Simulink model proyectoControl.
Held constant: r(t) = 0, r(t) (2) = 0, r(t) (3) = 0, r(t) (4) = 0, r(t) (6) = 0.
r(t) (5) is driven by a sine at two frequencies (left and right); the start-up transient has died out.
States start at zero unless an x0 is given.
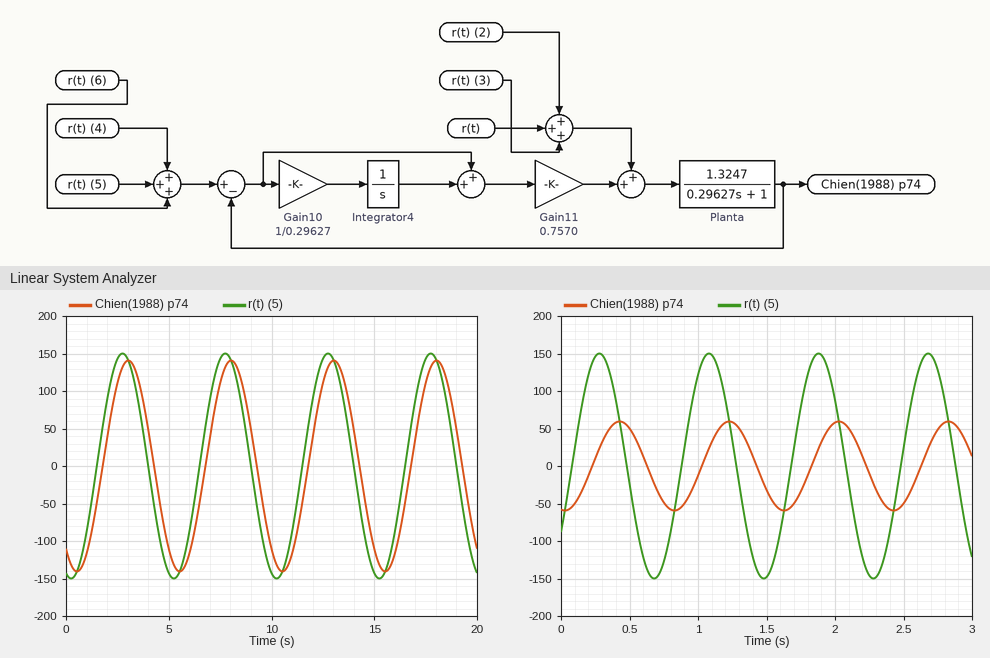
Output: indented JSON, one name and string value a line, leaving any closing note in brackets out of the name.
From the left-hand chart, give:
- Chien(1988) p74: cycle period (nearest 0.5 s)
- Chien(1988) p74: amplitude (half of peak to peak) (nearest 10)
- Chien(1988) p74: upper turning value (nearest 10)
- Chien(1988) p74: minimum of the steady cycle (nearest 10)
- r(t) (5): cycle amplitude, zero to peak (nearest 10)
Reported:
{
  "Chien(1988) p74: cycle period": "5.0 s",
  "Chien(1988) p74: amplitude (half of peak to peak)": "140",
  "Chien(1988) p74: upper turning value": "140",
  "Chien(1988) p74: minimum of the steady cycle": "-140",
  "r(t) (5): cycle amplitude, zero to peak": "150"
}
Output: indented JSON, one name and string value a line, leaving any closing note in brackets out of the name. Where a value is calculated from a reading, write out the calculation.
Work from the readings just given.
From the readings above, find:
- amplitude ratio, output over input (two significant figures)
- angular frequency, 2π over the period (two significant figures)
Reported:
{
  "amplitude ratio, output over input": "140 / 150 = 0.93",
  "angular frequency, 2π over the period": "2π / 5 = 1.3 rad/s"
}
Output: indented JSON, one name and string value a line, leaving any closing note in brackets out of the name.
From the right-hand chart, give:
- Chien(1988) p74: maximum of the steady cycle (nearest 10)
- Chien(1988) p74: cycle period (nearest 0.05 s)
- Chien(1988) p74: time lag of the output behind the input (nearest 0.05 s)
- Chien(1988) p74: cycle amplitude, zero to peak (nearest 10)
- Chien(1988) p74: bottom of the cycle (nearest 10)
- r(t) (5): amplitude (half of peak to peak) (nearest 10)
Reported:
{
  "Chien(1988) p74: maximum of the steady cycle": "60",
  "Chien(1988) p74: cycle period": "0.80 s",
  "Chien(1988) p74: time lag of the output behind the input": "0.15 s",
  "Chien(1988) p74: cycle amplitude, zero to peak": "60",
  "Chien(1988) p74: bottom of the cycle": "-60",
  "r(t) (5): amplitude (half of peak to peak)": "150"
}
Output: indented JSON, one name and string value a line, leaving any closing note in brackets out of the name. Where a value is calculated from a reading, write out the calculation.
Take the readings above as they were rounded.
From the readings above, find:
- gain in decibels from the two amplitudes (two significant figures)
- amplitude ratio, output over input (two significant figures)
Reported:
{
  "gain in decibels from the two amplitudes": "20 log10(60 / 150) = -8.0 dB",
  "amplitude ratio, output over input": "60 / 150 = 0.40"
}
